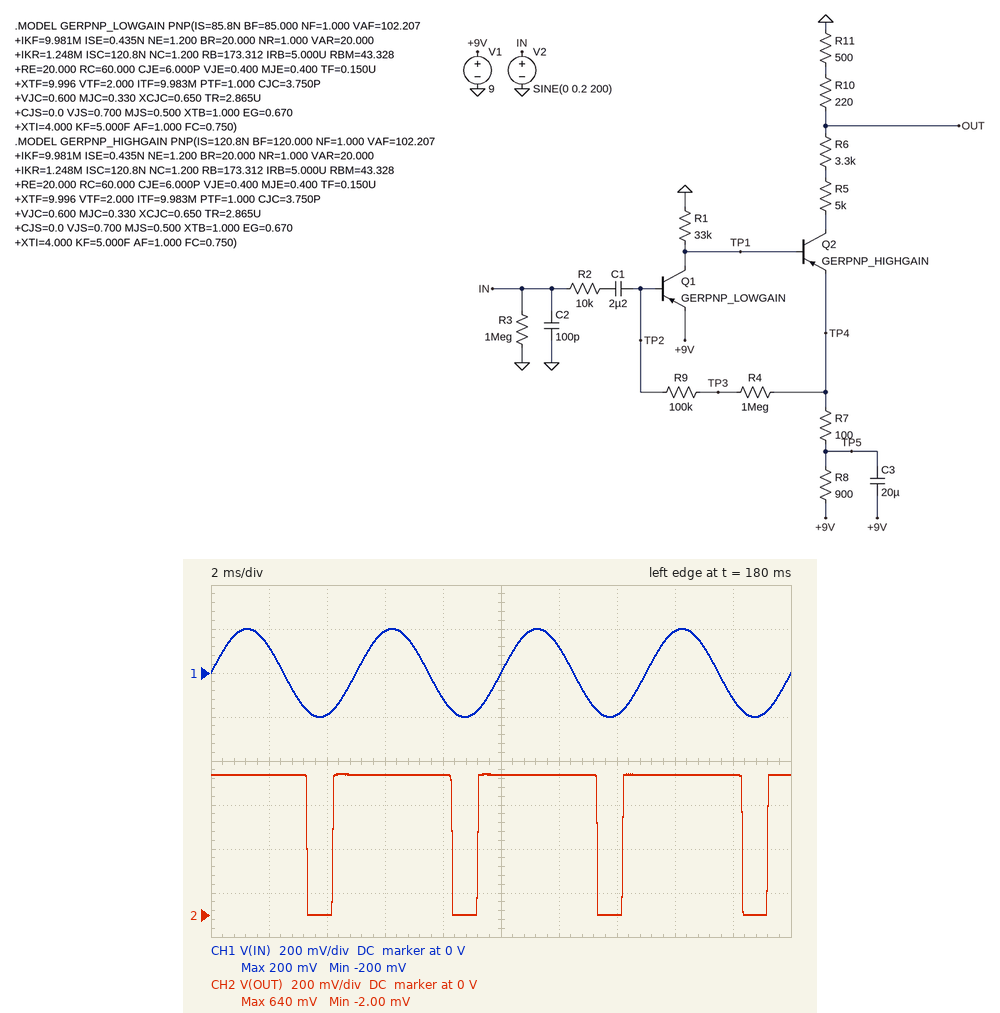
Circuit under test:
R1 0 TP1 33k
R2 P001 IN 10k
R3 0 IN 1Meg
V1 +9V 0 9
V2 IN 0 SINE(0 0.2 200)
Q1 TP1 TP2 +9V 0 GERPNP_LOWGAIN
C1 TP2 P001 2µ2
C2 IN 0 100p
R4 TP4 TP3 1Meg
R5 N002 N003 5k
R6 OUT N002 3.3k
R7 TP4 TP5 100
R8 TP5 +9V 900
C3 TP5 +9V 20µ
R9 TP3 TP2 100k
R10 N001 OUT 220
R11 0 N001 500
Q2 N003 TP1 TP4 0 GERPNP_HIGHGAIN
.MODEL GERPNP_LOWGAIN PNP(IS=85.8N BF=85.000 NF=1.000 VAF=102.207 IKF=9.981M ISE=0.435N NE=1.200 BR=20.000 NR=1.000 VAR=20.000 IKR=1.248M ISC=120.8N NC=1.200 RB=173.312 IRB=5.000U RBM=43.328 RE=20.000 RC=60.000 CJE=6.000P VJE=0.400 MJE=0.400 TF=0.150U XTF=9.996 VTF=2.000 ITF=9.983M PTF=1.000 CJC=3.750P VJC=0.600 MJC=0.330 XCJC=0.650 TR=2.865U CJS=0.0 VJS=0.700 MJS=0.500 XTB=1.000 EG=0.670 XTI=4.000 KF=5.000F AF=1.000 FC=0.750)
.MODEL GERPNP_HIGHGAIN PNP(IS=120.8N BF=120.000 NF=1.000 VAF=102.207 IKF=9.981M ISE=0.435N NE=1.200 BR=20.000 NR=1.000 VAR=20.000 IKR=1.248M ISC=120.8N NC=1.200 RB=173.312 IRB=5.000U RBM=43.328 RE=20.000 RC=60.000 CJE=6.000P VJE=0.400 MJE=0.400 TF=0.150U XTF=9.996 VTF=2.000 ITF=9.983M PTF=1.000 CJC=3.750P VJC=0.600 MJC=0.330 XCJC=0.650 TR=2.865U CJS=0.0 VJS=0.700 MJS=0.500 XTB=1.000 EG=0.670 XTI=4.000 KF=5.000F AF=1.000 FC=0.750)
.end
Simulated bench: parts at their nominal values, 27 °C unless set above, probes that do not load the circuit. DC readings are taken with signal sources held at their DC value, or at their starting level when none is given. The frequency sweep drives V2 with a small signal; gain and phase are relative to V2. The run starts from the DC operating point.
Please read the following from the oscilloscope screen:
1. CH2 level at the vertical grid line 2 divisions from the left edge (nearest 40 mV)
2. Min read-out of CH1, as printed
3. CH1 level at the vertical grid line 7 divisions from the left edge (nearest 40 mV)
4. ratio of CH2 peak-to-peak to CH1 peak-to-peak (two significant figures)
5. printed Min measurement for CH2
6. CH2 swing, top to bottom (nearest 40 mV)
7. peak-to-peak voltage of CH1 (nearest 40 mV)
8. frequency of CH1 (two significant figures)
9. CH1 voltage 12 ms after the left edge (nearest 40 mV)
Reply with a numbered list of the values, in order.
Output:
1. 0 V
2. -200 mV
3. -200 mV
4. 1.6
5. -2.00 mV
6. 640 mV
7. 400 mV
8. 200 Hz
9. 120 mV
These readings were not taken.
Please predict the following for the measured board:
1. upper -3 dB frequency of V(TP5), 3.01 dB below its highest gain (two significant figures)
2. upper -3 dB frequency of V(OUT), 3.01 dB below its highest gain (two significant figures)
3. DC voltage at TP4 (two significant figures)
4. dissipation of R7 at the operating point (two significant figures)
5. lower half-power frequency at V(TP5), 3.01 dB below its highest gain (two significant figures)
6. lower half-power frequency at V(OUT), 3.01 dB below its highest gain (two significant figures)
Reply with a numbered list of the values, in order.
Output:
1. 13 Hz
2. 13 Hz
3. 8.0 V
4. 110 µW
5. 1.4 Hz
6. 1.4 Hz
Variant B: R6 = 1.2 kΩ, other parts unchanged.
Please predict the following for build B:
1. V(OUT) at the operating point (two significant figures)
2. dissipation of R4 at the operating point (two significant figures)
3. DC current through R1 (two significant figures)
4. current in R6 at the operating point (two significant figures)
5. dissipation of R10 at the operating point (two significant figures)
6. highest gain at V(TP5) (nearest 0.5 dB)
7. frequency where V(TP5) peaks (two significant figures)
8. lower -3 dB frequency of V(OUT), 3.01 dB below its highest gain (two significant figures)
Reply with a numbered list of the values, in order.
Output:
1. 790 mV
2. 940 nW
3. 230 µA
4. 1.1 mA
5. 270 µW
6. 2.5 dB
7. 4.7 Hz
8. 1.6 Hz
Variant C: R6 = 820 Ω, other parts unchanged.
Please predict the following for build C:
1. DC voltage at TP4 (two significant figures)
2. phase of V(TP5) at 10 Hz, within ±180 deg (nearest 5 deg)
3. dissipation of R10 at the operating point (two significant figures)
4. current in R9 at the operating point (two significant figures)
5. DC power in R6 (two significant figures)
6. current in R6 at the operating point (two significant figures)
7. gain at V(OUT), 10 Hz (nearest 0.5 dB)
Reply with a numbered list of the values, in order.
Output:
1. 7.7 V
2. 150 deg
3. 290 µW
4. 1.0 µA
5. 1.1 mW
6. 1.2 mA
7. -18.5 dB
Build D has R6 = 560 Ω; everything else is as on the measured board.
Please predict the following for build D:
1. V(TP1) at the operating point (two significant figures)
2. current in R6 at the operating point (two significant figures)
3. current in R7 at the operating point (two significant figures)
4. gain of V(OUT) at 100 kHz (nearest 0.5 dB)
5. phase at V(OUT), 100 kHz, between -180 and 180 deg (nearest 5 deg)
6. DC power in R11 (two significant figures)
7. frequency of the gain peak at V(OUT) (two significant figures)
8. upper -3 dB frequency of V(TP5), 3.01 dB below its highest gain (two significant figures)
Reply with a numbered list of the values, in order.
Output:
1. 7.4 V
2. 1.2 mA
3. 1.3 mA
4. -37.0 dB
5. 125 deg
6. 720 µW
7. 4.8 Hz
8. 14 Hz
